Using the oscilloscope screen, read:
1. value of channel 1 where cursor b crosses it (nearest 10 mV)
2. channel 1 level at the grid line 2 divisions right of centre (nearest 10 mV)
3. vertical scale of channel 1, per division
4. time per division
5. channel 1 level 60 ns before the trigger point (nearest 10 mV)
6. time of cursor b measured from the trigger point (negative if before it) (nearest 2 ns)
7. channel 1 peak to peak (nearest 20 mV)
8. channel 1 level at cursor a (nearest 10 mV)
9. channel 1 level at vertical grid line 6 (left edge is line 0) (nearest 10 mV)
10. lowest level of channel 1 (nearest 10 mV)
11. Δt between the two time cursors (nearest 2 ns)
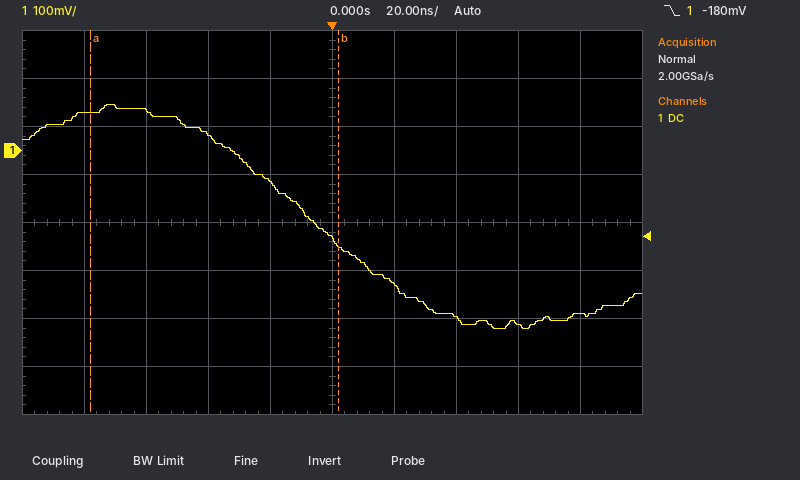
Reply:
-200 mV
-350 mV
100 mV
20 ns
80 mV
+2 ns
460 mV
80 mV
-280 mV
-370 mV
80 ns
